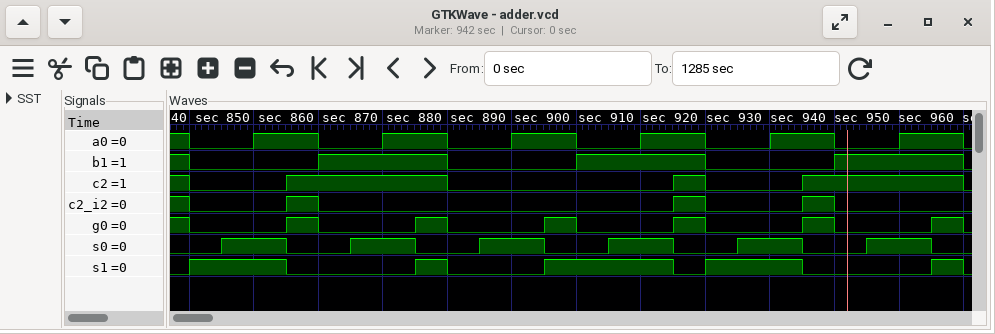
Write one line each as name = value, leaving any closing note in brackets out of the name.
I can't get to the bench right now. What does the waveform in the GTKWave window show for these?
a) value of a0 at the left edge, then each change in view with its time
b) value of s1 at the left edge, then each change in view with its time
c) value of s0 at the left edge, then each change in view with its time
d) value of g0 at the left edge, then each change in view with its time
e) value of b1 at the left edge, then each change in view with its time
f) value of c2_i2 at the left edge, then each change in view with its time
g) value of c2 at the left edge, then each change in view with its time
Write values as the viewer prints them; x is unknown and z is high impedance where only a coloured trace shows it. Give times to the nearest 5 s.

value of a0 at the left edge, then each change in view with its time = 1, 0 at 840 s, 1 at 850 s, 0 at 860 s, 1 at 870 s, 0 at 880 s, 1 at 890 s, 0 at 900 s, 1 at 910 s, 0 at 920 s, 1 at 930 s, 0 at 940 s, 1 at 950 s, 0 at 960 s
value of s1 at the left edge, then each change in view with its time = 0, 1 at 840 s, 0 at 855 s, 1 at 875 s, 0 at 880 s, 1 at 895 s, 0 at 915 s, 1 at 920 s, 0 at 935 s, 1 at 955 s, 0 at 960 s
value of s0 at the left edge, then each change in view with its time = 0, 1 at 845 s, 0 at 855 s, 1 at 865 s, 0 at 875 s, 1 at 885 s, 0 at 895 s, 1 at 905 s, 0 at 915 s, 1 at 925 s, 0 at 935 s, 1 at 945 s, 0 at 955 s
value of g0 at the left edge, then each change in view with its time = 1, 0 at 840 s, 1 at 855 s, 0 at 860 s, 1 at 875 s, 0 at 880 s, 1 at 895 s, 0 at 900 s, 1 at 915 s, 0 at 920 s, 1 at 935 s, 0 at 940 s, 1 at 955 s, 0 at 960 s
value of b1 at the left edge, then each change in view with its time = 1, 0 at 840 s, 1 at 860 s, 0 at 880 s, 1 at 900 s, 0 at 920 s, 1 at 940 s, 0 at 960 s
value of c2_i2 at the left edge, then each change in view with its time = 1, 0 at 840 s, 1 at 855 s, 0 at 860 s, 1 at 915 s, 0 at 920 s, 1 at 935 s, 0 at 940 s
value of c2 at the left edge, then each change in view with its time = 1, 0 at 840 s, 1 at 855 s, 0 at 880 s, 1 at 915 s, 0 at 920 s, 1 at 935 s, 0 at 960 s
